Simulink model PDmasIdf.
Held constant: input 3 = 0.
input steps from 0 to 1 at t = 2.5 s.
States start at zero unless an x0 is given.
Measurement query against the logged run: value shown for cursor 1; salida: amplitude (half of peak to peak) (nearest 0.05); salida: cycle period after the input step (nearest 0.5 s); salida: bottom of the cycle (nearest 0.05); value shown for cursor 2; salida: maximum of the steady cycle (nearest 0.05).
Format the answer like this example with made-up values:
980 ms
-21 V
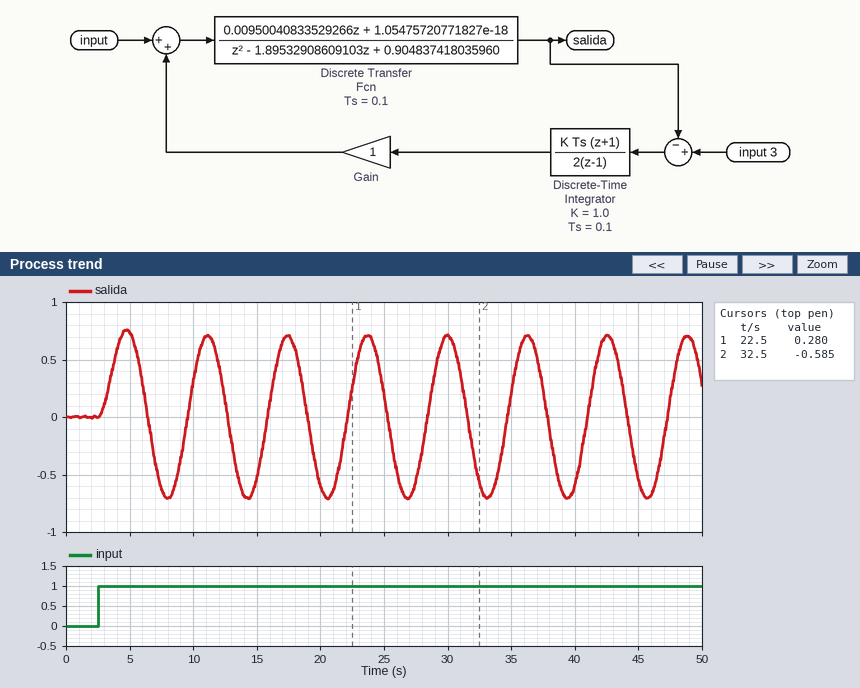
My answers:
0.280
0.70
6.5 s
-0.70
-0.585
0.70
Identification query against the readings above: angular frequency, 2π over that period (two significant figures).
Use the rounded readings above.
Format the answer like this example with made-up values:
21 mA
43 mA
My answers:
0.97 rad/s
